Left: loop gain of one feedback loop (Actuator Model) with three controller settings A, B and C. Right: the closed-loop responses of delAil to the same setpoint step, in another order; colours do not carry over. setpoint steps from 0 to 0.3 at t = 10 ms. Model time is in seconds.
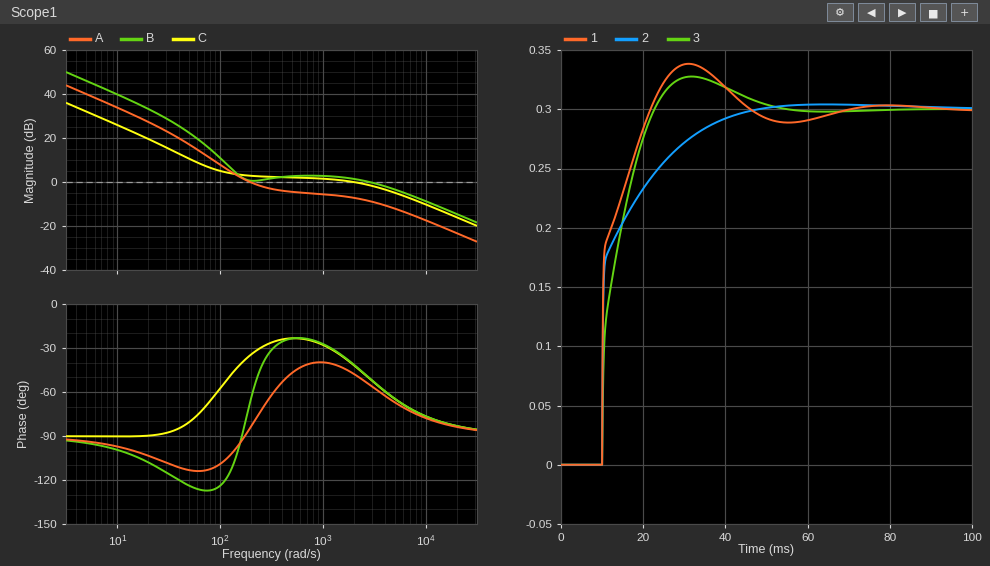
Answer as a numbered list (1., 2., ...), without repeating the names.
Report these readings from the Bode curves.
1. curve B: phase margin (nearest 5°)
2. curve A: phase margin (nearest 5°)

1. 130°
2. 95°
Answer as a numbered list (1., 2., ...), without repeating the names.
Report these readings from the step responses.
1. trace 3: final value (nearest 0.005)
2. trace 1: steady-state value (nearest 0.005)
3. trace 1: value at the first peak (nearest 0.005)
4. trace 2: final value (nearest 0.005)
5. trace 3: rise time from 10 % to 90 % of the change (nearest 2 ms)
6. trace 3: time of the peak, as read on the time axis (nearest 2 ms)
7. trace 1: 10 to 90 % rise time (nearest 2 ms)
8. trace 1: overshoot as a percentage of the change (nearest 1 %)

1. 0.300
2. 0.300
3. 0.340
4. 0.300
5. 10 ms
6. 32 ms
7. 8 ms
8. 13 %
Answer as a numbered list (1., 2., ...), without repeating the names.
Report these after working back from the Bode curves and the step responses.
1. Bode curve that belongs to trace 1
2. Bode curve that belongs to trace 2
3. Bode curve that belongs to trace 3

1. B
2. C
3. A
